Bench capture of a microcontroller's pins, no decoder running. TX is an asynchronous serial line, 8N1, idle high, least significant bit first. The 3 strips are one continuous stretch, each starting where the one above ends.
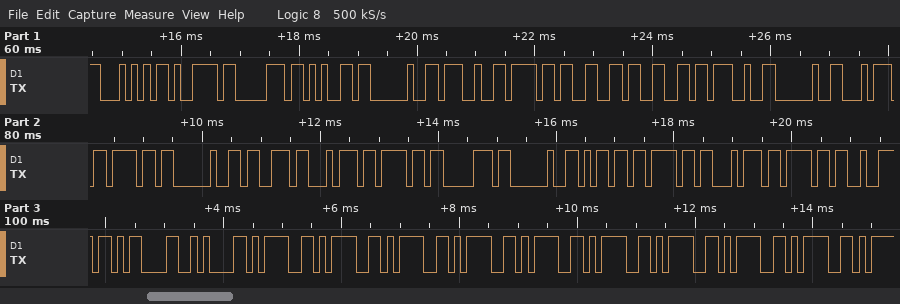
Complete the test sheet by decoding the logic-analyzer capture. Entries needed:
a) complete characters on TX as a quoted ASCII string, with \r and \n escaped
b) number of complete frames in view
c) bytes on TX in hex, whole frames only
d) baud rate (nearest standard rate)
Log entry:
"Type 'off' to stop motor\r\n========="
35
0x54 0x79 0x70 0x65 0x20 0x27 0x6F 0x66 0x66 0x27 0x20 0x74 0x6F 0x20 0x73 0x74 0x6F 0x70 0x20 0x6D 0x6F 0x74 0x6F 0x72 0x0D 0x0A 0x3D 0x3D 0x3D 0x3D 0x3D 0x3D 0x3D 0x3D 0x3D
9600 baud
